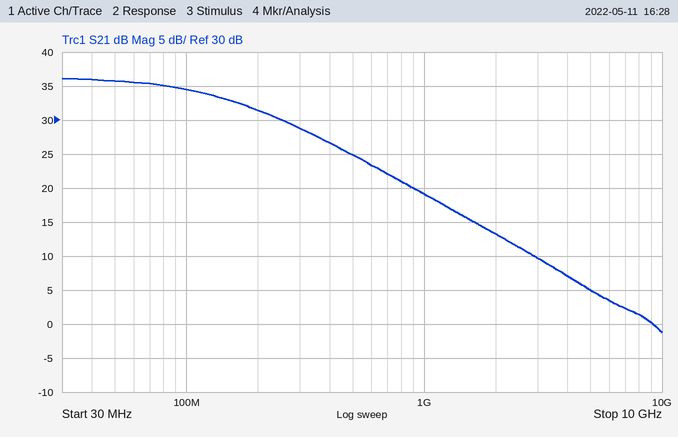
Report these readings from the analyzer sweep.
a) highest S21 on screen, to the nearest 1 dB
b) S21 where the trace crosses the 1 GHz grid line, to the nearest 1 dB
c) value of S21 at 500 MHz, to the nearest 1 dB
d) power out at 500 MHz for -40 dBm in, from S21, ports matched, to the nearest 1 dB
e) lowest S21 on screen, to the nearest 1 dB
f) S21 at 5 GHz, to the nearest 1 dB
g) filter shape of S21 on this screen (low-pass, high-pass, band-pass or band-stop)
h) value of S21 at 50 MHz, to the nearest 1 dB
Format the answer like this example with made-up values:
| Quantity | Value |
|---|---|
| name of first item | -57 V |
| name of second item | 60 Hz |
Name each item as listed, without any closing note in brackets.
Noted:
| Quantity | Value |
|---|---|
| highest S21 on screen, to the nearest 1 dB | 36 dB |
| S21 where the trace crosses the 1 GHz grid line, to the nearest 1 dB | 19 dB |
| value of S21 at 500 MHz, to the nearest 1 dB | 25 dB |
| power out at 500 MHz for -40 dBm in, from S21, ports matched, to the nearest 1 dB | -15 dBm |
| lowest S21 on screen, to the nearest 1 dB | -1 dB |
| S21 at 5 GHz, to the nearest 1 dB | 5 dB |
| filter shape of S21 on this screen | low-pass |
| value of S21 at 50 MHz, to the nearest 1 dB | 36 dB |
